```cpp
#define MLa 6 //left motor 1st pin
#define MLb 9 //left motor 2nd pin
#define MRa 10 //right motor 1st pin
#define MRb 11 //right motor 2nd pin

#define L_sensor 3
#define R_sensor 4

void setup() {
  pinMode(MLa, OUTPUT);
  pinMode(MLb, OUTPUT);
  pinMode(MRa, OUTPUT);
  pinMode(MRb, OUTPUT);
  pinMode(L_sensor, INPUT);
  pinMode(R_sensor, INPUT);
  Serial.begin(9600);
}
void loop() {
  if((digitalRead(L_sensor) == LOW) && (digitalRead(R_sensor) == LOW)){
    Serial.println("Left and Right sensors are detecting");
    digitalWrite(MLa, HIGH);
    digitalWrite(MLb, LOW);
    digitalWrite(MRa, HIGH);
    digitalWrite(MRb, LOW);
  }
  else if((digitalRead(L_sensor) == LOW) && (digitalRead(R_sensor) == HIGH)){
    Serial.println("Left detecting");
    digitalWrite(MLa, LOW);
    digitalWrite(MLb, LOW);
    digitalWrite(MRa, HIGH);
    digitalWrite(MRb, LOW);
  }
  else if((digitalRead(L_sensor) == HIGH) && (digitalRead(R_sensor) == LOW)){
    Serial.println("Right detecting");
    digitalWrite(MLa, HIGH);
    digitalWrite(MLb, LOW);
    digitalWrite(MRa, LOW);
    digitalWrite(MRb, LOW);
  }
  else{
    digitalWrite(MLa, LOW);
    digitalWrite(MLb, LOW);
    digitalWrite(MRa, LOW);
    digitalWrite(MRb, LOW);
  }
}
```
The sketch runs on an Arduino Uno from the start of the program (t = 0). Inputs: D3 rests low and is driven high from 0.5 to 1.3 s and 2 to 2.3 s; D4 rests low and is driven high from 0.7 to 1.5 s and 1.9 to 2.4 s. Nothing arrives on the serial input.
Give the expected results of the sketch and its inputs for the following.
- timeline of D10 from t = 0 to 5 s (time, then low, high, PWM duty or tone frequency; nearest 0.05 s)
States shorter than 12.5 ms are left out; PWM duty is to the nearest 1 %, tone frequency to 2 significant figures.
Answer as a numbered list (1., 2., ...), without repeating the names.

1. 0 s high; 0.55 s low; 1.3 s high; 2 s low; 2.3 s high
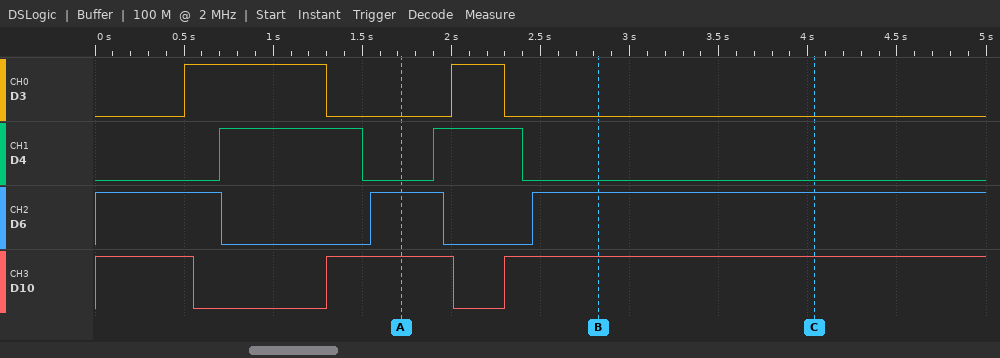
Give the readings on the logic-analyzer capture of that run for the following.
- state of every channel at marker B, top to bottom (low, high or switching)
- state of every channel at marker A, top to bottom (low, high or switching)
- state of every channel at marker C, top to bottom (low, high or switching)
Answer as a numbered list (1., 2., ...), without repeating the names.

1. D3 low, D4 low, D6 high, D10 high
2. D3 low, D4 low, D6 high, D10 high
3. D3 low, D4 low, D6 high, D10 high
